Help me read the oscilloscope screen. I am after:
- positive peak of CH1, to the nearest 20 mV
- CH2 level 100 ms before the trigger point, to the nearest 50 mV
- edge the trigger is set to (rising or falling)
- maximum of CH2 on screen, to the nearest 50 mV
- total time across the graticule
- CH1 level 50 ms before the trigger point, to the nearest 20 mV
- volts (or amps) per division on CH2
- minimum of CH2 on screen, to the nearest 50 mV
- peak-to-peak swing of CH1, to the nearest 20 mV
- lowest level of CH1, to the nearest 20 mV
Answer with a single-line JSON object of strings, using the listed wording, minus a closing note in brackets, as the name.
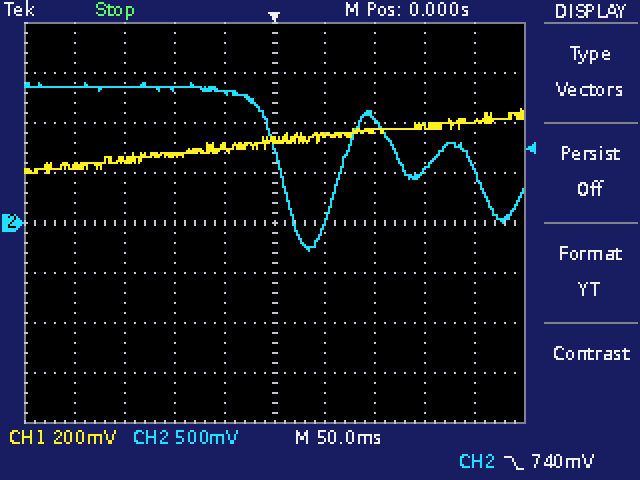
{"positive peak of CH1, to the nearest 20 mV": "460 mV", "CH2 level 100 ms before the trigger point, to the nearest 50 mV": "1.35 V", "edge the trigger is set to": "falling", "maximum of CH2 on screen, to the nearest 50 mV": "1.40 V", "total time across the graticule": "500 ms", "CH1 level 50 ms before the trigger point, to the nearest 20 mV": "300 mV", "volts (or amps) per division on CH2": "500 mV", "minimum of CH2 on screen, to the nearest 50 mV": "-300 mV", "peak-to-peak swing of CH1, to the nearest 20 mV": "260 mV", "lowest level of CH1, to the nearest 20 mV": "200 mV"}
